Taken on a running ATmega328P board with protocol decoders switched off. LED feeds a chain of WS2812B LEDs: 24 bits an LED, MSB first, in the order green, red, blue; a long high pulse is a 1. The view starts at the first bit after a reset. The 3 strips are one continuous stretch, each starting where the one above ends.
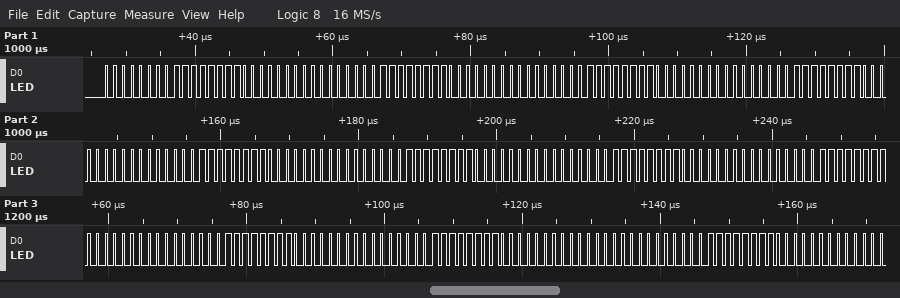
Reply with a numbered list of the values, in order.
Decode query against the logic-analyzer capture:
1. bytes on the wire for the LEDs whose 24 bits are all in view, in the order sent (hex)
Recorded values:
1. 00 FF 00 00 FF 00 00 FF 00 00 FF 00 00 FF 00 00 FF 00 00 FF 00 00 FF 00 00 FF 00 00 FF 00 00 00 FF
